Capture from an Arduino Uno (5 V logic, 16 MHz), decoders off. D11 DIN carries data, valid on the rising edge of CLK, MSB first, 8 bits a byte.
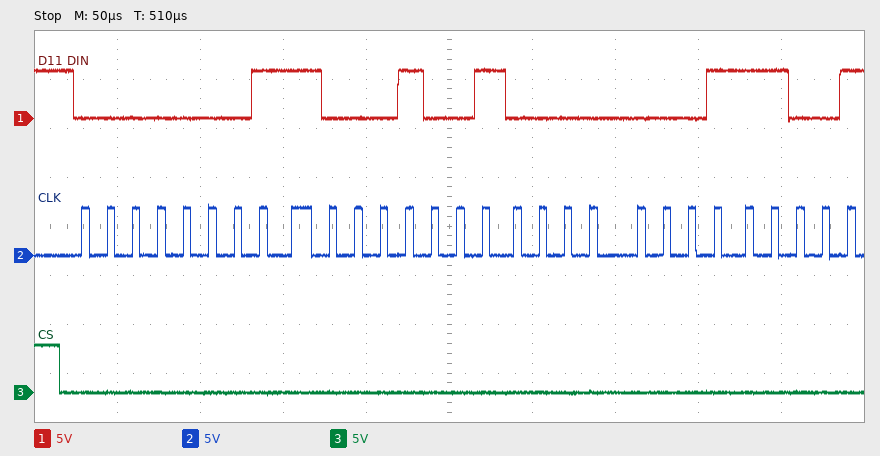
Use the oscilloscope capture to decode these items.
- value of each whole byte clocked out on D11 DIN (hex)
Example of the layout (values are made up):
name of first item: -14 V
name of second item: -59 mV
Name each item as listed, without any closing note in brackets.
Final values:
value of each whole byte clocked out on D11 DIN: 01 89 01
